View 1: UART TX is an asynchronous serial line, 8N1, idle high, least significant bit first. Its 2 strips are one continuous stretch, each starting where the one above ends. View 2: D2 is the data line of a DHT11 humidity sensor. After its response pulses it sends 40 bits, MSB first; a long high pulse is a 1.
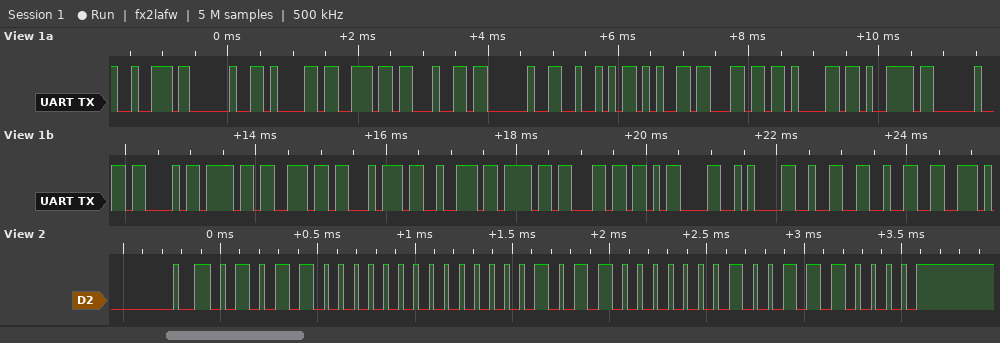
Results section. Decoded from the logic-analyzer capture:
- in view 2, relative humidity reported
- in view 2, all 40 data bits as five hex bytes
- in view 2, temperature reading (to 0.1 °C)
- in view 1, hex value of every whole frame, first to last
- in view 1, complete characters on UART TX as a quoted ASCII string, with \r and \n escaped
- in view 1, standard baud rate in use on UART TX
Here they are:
88 %
58 00 16 02 70
22.2 °C
72 20 61 6E 64 20 52 65 6C 61 79 20 43 6F 6E 74 72 6F 6C 0D 0A 32 32
"r and Relay Control\r\n22"
9600 baud
